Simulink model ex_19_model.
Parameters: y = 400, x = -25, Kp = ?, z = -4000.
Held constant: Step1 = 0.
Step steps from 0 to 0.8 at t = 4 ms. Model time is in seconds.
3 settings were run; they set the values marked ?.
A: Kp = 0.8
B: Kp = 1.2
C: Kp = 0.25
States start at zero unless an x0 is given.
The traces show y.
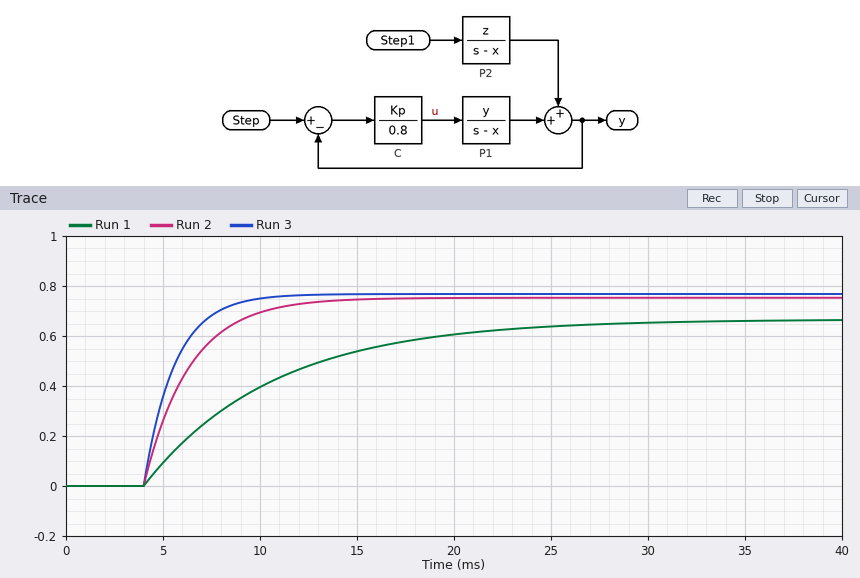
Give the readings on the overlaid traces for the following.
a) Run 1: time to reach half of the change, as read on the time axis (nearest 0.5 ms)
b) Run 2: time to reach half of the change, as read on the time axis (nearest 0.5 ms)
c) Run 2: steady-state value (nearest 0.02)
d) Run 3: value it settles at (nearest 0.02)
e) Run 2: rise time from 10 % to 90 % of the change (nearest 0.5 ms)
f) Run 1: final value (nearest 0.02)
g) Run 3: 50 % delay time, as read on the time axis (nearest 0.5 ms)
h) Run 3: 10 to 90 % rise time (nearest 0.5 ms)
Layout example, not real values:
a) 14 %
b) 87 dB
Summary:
a) 8.5 ms
b) 5.5 ms
c) 0.76
d) 0.76
e) 5.0 ms
f) 0.66
g) 5.0 ms
h) 3.5 ms
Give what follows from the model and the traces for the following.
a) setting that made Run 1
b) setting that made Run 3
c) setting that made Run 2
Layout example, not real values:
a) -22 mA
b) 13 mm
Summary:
a) C
b) B
c) A
